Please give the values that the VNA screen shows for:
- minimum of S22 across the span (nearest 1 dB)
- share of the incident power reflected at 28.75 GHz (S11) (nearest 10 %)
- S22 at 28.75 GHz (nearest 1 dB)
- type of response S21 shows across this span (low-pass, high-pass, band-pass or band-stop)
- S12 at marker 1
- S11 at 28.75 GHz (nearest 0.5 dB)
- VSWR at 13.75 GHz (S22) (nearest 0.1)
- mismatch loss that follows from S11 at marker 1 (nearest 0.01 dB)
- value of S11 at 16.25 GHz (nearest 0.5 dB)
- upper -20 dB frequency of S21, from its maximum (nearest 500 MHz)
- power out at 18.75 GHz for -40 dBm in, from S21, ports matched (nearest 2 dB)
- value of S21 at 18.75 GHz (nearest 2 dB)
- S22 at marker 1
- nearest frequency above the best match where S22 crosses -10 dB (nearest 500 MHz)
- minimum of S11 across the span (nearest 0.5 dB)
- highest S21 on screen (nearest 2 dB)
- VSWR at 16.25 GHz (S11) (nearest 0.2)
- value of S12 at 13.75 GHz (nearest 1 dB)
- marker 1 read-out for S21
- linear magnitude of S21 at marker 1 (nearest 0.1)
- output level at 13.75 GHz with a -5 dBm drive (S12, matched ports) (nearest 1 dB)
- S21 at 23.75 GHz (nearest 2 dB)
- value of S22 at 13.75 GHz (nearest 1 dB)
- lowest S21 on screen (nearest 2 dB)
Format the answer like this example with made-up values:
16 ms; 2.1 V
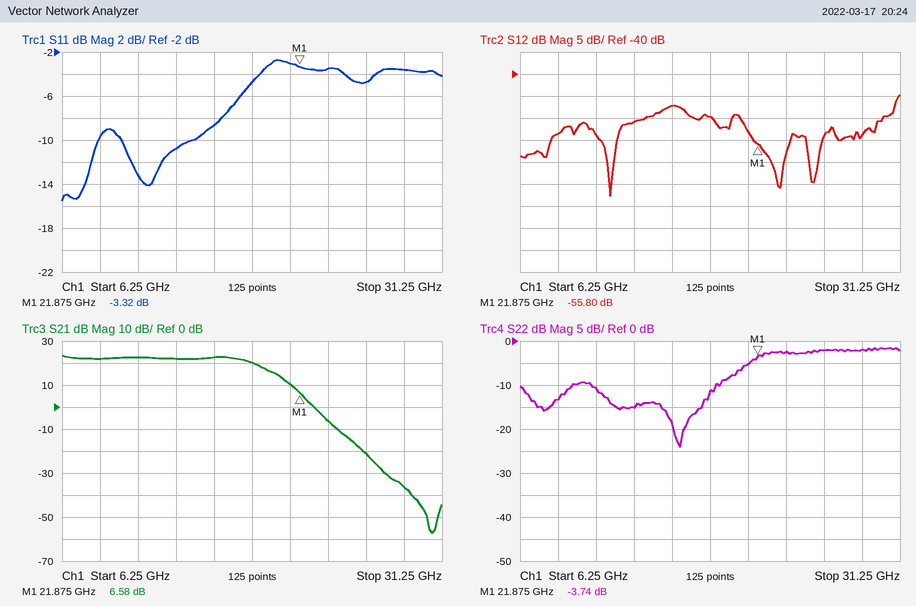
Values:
-24 dB; 40 %; -2 dB; low-pass; -55.80 dB; -3.5 dB; 1.4; 2.72 dB; -8.5 dB; 22.5 GHz; -20 dBm; 20 dB; -3.74 dB; 19.0 GHz; -15.5 dB; 24 dB; 2.2; -51 dB; 6.58 dB; 2.1; -56 dBm; -6 dB; -15 dB; -58 dB
